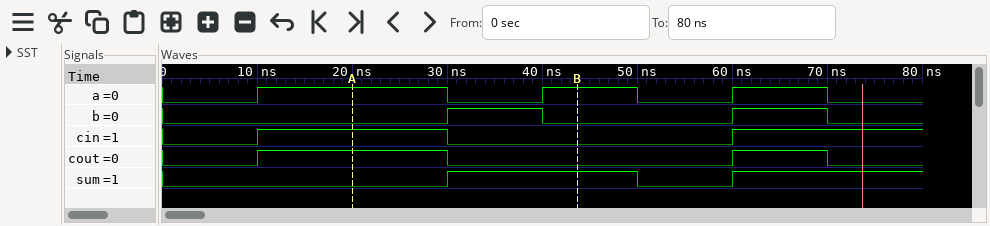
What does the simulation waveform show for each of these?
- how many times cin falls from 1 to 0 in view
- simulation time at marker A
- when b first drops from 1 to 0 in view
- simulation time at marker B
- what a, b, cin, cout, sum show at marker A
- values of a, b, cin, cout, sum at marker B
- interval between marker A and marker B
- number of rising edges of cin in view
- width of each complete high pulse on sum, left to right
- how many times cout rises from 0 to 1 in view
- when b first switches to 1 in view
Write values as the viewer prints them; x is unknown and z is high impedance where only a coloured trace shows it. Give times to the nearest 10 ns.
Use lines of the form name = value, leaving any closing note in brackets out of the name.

how many times cin falls from 1 to 0 in view = 1
simulation time at marker A = 20 ns
when b first drops from 1 to 0 in view = 40 ns
simulation time at marker B = 40 ns
what a, b, cin, cout, sum show at marker A = a=1, b=0, cin=1, cout=1, sum=0
values of a, b, cin, cout, sum at marker B = a=1, b=0, cin=0, cout=0, sum=1
interval between marker A and marker B = 20 ns
number of rising edges of cin in view = 2
width of each complete high pulse on sum, left to right = 20 ns
how many times cout rises from 0 to 1 in view = 2
when b first switches to 1 in view = 30 ns
